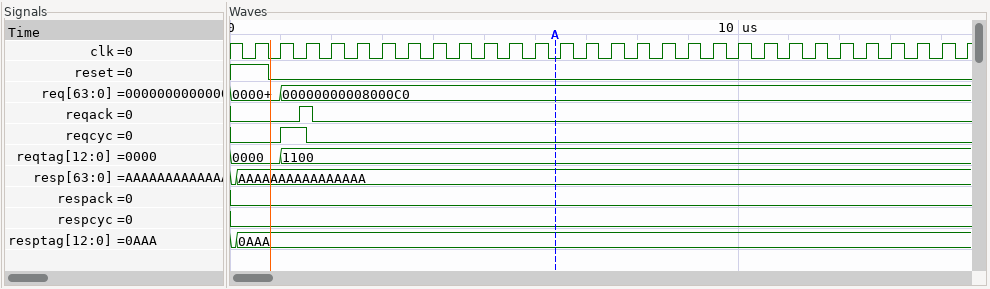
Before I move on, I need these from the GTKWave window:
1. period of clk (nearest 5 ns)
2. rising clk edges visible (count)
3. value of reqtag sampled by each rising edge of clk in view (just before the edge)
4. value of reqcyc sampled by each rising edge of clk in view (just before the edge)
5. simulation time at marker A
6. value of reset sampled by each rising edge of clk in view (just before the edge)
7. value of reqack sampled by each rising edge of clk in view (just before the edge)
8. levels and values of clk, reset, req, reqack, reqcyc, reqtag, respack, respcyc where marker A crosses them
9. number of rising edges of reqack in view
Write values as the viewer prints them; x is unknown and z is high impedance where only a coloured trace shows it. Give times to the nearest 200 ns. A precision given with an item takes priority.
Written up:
500 ns
29
0000, 0000, 1100, 1100, 1100, 1100, 1100, 1100, 1100, 1100, 1100, 1100, 1100, 1100, 1100, 1100, 1100, 1100, 1100, 1100, 1100, 1100, 1100, 1100, 1100, 1100, 1100, 1100, 1100
0 0 1 0 0 0 0 0 0 0 0 0 0 0 0 0 0 0 0 0 0 0 0 0 0 0 0 0 0
6400 ns
1 0 0 0 0 0 0 0 0 0 0 0 0 0 0 0 0 0 0 0 0 0 0 0 0 0 0 0 0
0 0 1 0 0 0 0 0 0 0 0 0 0 0 0 0 0 0 0 0 0 0 0 0 0 0 0 0 0
clk=0, reset=0, req=00000000008000C0, reqack=0, reqcyc=0, reqtag=1100, respack=0, respcyc=0
1
